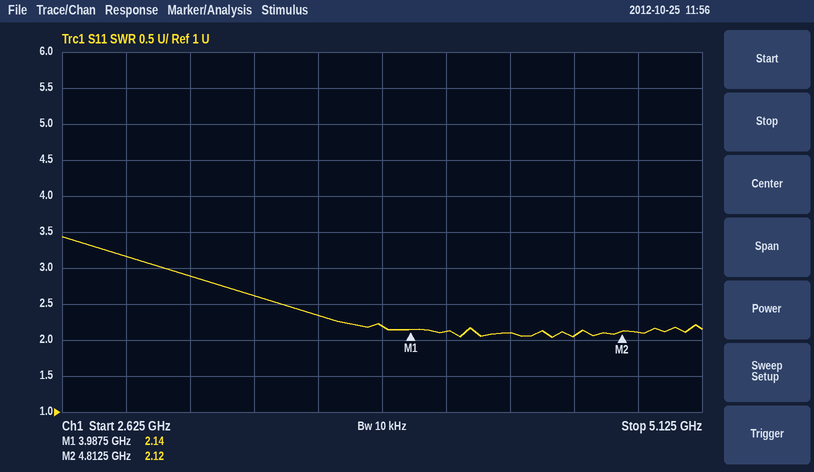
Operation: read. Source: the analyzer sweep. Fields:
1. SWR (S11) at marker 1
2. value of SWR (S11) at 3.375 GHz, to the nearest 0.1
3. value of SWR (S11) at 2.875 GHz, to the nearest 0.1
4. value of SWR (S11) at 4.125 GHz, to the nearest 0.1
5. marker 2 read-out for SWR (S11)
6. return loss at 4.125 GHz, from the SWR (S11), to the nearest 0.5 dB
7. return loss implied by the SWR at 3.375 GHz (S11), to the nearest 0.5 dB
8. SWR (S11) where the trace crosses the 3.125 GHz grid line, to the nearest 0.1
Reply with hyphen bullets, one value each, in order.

- 2.14
- 2.6
- 3.2
- 2.1
- 2.12
- 9.0 dB
- 7.0 dB
- 2.9
